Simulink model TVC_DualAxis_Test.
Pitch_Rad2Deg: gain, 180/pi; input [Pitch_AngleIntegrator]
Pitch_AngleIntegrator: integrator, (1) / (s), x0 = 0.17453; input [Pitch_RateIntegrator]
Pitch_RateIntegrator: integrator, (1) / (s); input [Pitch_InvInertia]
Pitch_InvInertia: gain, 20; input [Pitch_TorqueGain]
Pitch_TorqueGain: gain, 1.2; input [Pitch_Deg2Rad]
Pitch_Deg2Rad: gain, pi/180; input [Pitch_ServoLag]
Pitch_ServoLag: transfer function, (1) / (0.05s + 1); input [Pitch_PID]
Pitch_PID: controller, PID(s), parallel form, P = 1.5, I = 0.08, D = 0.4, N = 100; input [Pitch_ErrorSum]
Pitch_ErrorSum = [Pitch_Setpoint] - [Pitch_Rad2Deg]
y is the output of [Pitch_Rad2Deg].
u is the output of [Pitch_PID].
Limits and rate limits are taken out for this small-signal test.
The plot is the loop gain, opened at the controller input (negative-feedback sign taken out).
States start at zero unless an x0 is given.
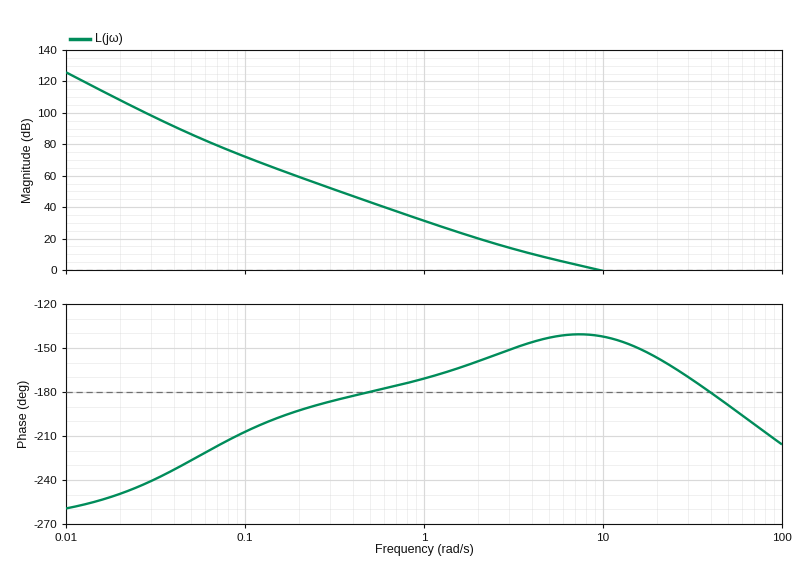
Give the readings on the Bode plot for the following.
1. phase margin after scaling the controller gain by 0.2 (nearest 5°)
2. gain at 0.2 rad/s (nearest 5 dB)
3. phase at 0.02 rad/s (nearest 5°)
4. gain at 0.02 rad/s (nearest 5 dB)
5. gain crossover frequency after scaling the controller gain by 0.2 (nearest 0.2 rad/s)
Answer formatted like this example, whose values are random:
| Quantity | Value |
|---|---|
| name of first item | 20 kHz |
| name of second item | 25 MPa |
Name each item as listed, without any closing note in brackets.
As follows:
| Quantity | Value |
|---|---|
| phase margin after scaling the controller gain by 0.2 | 30° |
| gain at 0.2 rad/s | 60 dB |
| phase at 0.02 rad/s | -250° |
| gain at 0.02 rad/s | 110 dB |
| gain crossover frequency after scaling the controller gain by 0.2 | 3.0 rad/s |
